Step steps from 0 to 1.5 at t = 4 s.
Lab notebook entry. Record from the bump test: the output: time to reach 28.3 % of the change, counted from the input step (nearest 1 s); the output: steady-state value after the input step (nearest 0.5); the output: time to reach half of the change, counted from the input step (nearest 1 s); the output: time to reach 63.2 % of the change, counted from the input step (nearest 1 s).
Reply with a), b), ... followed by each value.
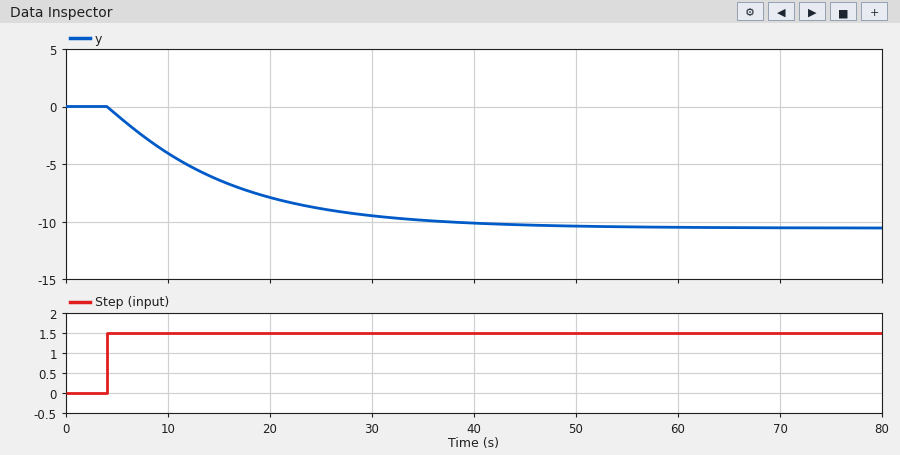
a) 4 s
b) -10.5
c) 8 s
d) 12 s
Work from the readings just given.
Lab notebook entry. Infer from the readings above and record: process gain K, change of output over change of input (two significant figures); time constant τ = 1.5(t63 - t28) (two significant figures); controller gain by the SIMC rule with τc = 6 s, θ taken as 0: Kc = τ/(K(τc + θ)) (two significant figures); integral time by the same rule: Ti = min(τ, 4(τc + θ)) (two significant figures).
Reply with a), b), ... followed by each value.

a) -7.0
b) 12 s
c) -0.29
d) 12 s
